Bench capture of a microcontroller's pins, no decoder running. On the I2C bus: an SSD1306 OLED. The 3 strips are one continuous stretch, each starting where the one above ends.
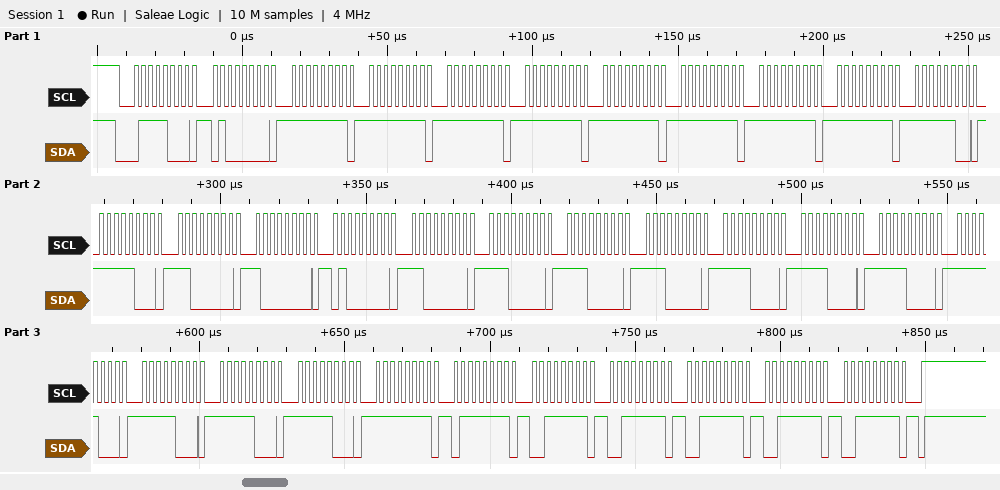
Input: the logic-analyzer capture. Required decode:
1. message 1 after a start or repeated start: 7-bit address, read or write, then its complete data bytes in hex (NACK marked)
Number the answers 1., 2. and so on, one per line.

1. 0x3C write: 40 FF FF FF FF FF FF FF FF FC F8 C0 80 40 C0 E0 E0 E0 F0 F0 F0 F8 F8 F8 F8 FF 7F 3F 3F 3F 3F 3F
